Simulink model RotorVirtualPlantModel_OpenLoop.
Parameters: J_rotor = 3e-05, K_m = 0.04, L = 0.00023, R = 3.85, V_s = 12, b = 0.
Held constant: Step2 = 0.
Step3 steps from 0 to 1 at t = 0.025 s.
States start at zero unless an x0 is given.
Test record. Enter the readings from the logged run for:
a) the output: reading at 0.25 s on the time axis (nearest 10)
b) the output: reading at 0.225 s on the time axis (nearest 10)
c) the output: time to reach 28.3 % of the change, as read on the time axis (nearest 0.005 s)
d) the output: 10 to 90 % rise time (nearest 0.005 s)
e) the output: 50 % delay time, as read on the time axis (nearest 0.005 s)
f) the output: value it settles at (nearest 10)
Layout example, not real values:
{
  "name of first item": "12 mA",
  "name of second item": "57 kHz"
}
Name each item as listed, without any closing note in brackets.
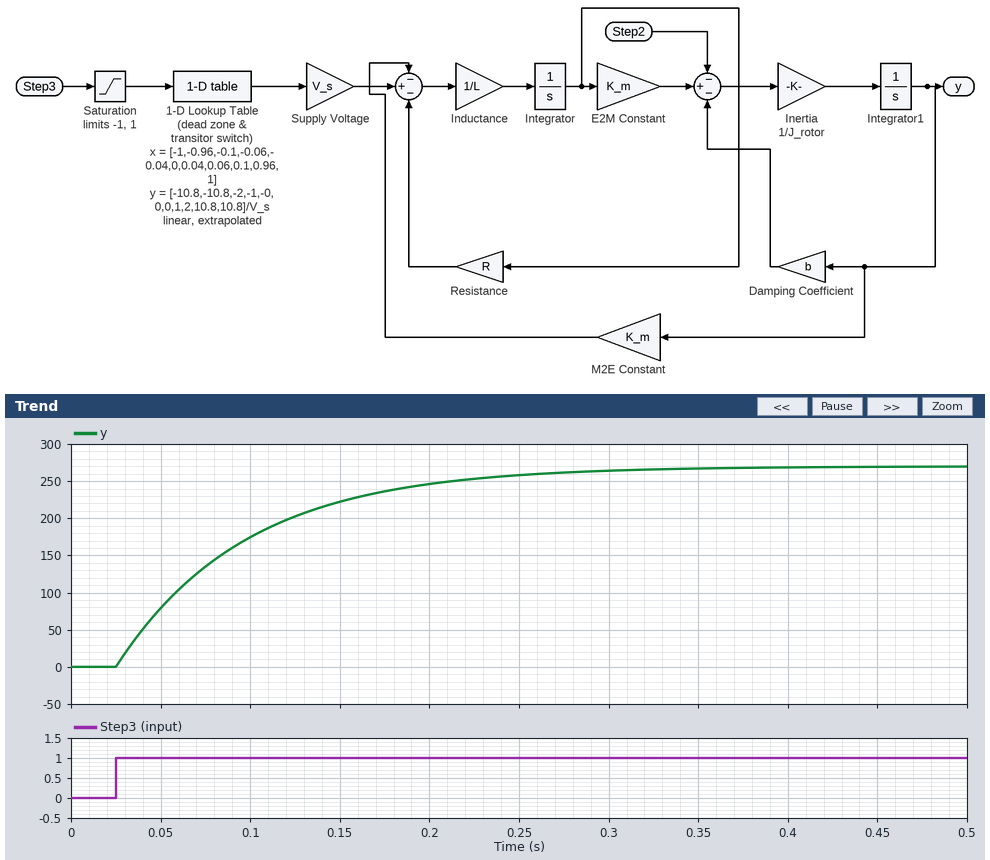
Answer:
{
  "the output: reading at 0.25 s on the time axis": "260",
  "the output: reading at 0.225 s on the time axis": "250",
  "the output: time to reach 28.3 % of the change, as read on the time axis": "0.050 s",
  "the output: 10 to 90 % rise time": "0.160 s",
  "the output: 50 % delay time, as read on the time axis": "0.075 s",
  "the output: value it settles at": "270"
}
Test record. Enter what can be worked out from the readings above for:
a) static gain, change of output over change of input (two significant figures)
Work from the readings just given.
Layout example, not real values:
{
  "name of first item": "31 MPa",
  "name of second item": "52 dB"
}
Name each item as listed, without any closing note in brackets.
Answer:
{
  "static gain, change of output over change of input": "270"
}
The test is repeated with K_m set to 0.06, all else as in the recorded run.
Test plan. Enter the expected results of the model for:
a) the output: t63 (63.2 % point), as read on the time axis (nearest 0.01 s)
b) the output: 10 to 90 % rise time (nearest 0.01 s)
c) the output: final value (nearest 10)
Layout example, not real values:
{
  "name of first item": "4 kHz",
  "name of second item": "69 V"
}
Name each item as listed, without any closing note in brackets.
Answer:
{
  "the output: t63 (63.2 % point), as read on the time axis": "0.06 s",
  "the output: 10 to 90 % rise time": "0.07 s",
  "the output: final value": "180"
}
